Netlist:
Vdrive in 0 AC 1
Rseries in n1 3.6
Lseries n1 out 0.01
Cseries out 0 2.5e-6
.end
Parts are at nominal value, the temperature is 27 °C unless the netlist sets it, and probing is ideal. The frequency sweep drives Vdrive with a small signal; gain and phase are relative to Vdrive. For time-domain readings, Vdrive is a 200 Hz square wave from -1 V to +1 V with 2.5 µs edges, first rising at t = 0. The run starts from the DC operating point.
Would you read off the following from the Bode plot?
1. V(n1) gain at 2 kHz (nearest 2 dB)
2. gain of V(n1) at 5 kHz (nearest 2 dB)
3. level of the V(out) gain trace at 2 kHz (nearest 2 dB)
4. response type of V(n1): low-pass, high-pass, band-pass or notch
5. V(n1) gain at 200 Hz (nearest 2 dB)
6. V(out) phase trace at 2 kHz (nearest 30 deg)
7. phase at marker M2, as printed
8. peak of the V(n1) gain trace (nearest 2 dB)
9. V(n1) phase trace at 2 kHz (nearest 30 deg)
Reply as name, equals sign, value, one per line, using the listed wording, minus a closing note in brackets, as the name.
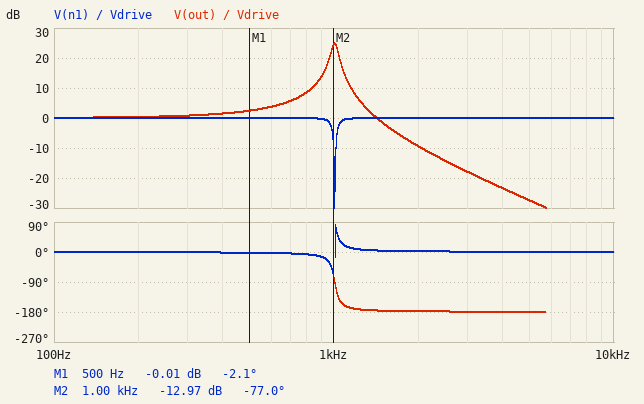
V(n1) gain at 2 kHz = 0 dB
gain of V(n1) at 5 kHz = 0 dB
level of the V(out) gain trace at 2 kHz = -10 dB
response type of V(n1): low-pass, high-pass, band-pass or notch = notch
V(n1) gain at 200 Hz = 0 dB
V(out) phase trace at 2 kHz = -180 deg
phase at marker M2, as printed = -77.0 deg
peak of the V(n1) gain trace = 0 dB
V(n1) phase trace at 2 kHz = 0 deg
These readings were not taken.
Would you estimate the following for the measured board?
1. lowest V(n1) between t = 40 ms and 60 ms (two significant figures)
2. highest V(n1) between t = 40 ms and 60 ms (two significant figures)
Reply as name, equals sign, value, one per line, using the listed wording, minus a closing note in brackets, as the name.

lowest V(n1) between t = 40 ms and 60 ms = -1.3 V
highest V(n1) between t = 40 ms and 60 ms = 1.3 V
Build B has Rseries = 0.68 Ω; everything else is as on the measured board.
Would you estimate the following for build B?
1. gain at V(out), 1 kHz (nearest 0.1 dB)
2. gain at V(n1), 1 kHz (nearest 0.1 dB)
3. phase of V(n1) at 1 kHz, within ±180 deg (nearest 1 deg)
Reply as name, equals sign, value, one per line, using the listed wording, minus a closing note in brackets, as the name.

gain at V(out), 1 kHz = 35.5 dB
gain at V(n1), 1 kHz = -2.2 dB
phase of V(n1) at 1 kHz, within ±180 deg = -39 deg
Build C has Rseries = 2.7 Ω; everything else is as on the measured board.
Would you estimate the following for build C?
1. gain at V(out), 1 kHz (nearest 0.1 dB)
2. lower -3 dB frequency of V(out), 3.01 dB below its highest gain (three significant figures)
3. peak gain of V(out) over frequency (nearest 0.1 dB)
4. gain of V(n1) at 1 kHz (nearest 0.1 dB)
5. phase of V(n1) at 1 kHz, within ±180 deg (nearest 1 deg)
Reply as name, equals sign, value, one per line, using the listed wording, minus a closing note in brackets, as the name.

gain at V(out), 1 kHz = 27.1 dB
lower -3 dB frequency of V(out), 3.01 dB below its highest gain = 984 Hz
peak gain of V(out) over frequency = 27.4 dB
gain of V(n1) at 1 kHz = -10.6 dB
phase of V(n1) at 1 kHz, within ±180 deg = -73 deg
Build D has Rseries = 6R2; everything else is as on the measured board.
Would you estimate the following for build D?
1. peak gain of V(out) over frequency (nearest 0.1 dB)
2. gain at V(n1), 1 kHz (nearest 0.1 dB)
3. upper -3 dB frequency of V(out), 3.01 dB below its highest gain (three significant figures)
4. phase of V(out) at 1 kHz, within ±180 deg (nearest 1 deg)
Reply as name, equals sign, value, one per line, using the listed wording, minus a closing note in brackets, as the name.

peak gain of V(out) over frequency = 20.2 dB
gain at V(n1), 1 kHz = -17.5 dB
upper -3 dB frequency of V(out), 3.01 dB below its highest gain = 1.05 kHz
phase of V(out) at 1 kHz, within ±180 deg = -82 deg
